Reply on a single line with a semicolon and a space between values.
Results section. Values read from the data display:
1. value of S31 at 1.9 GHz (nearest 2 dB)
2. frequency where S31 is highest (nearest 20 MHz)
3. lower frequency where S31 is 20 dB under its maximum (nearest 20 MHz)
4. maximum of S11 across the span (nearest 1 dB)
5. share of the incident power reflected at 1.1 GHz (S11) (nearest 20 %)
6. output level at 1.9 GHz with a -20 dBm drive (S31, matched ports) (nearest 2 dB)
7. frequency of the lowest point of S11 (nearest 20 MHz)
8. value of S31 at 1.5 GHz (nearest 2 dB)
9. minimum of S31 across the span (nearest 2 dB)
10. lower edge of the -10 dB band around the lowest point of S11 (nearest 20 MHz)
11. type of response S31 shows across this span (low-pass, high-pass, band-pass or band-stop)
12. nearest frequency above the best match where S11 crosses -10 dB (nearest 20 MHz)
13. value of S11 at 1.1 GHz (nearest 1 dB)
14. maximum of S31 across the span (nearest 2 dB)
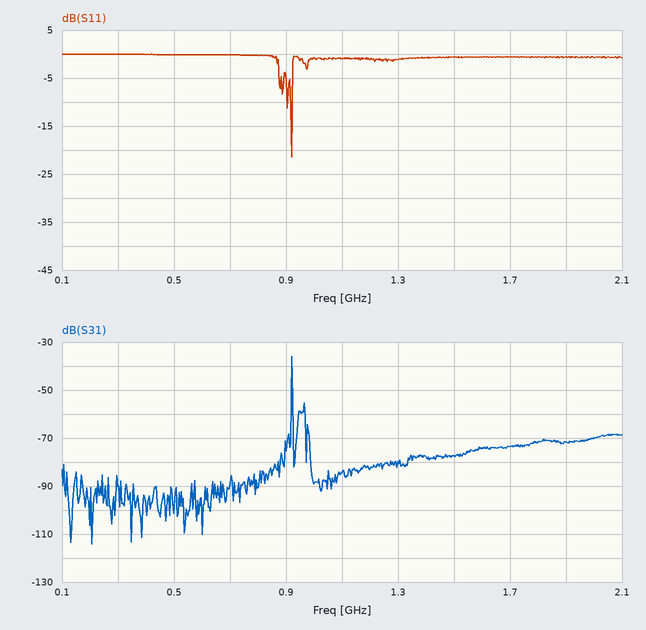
-72 dB; 920 MHz; 920 MHz; 0 dB; 80 %; -92 dBm; 920 MHz; -78 dB; -114 dB; 920 MHz; band-pass; 920 MHz; -1 dB; -36 dB
